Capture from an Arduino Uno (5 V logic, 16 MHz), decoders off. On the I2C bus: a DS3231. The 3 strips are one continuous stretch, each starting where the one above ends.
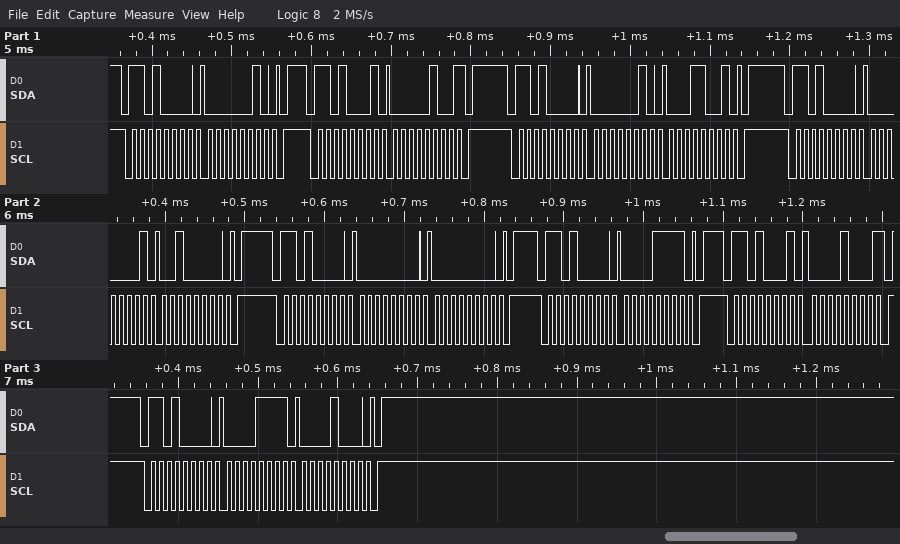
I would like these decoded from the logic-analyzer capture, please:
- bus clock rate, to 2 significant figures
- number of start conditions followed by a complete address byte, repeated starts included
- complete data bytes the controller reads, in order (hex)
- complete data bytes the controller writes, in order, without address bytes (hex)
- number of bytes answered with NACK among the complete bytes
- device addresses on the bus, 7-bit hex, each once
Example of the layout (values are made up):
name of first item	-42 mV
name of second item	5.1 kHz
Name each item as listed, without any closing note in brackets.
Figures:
bus clock rate, to 2 significant figures	100 kHz
number of start conditions followed by a complete address byte, repeated starts included	8
complete data bytes the controller reads, in order	04 08
complete data bytes the controller writes, in order, without address bytes	02 02 19 01 20 00 00 0F 0F 08
number of bytes answered with NACK among the complete bytes	2
device addresses on the bus, 7-bit hex, each once	0x68
